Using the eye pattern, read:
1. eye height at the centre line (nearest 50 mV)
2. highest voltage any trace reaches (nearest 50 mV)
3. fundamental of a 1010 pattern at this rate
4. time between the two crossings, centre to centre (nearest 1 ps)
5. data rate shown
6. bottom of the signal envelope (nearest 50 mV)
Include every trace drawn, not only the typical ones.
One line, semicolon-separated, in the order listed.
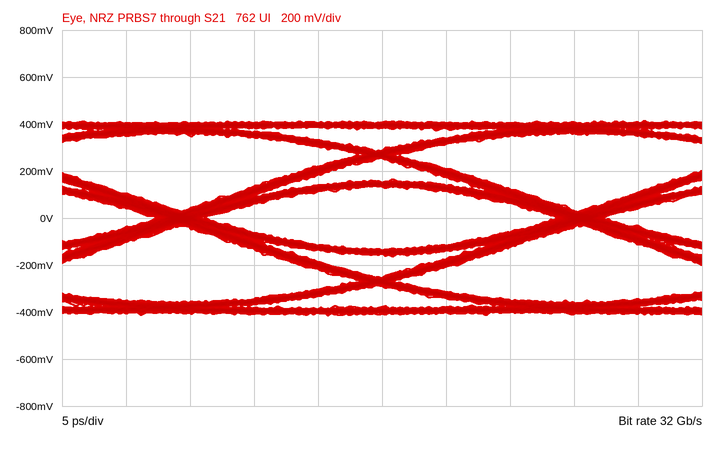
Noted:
250 mV; 400 mV; 16 GHz; 31 ps; 32 Gb/s; -400 mV
